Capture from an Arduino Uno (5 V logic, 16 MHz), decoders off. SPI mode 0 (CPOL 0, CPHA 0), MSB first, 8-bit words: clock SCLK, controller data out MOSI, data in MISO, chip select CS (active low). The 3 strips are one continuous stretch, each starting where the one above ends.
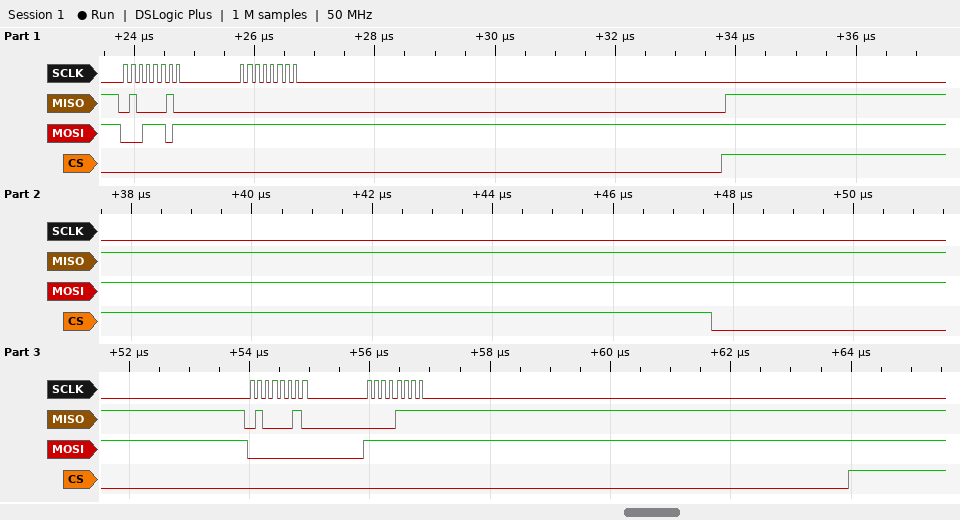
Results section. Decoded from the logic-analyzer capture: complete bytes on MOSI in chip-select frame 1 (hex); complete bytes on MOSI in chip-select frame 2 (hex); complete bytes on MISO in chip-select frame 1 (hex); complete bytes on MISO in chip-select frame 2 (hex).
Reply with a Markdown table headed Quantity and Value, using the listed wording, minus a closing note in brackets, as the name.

| Quantity | Value |
|---|---|
| complete bytes on MOSI in chip-select frame 1 | 1D FF |
| complete bytes on MOSI in chip-select frame 2 | 00 FF |
| complete bytes on MISO in chip-select frame 1 | 42 00 |
| complete bytes on MISO in chip-select frame 2 | 42 0F |
